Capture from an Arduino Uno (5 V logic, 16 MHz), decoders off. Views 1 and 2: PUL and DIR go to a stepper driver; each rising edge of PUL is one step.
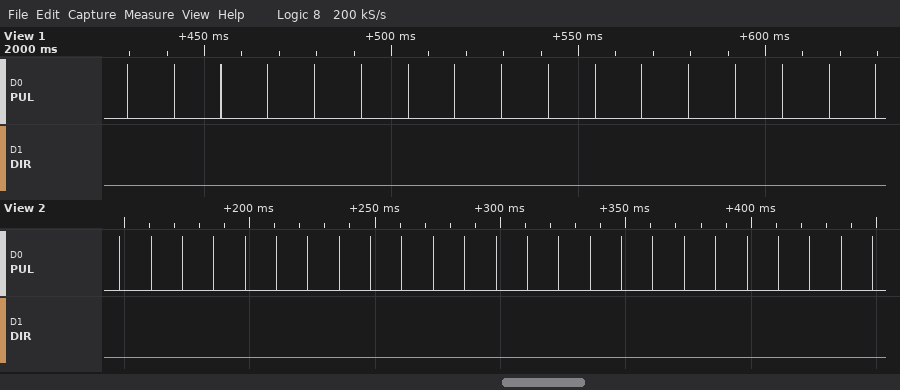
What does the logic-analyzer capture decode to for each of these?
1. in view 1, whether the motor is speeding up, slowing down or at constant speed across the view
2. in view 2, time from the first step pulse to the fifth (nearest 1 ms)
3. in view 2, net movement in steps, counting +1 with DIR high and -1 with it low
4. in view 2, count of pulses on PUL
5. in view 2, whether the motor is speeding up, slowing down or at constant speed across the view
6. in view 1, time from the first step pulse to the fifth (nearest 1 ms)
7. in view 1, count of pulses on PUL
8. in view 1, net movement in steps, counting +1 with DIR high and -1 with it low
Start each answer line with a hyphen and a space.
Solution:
- constant speed
- 50 ms
- -25
- 25
- constant speed
- 50 ms
- 17
- -17
